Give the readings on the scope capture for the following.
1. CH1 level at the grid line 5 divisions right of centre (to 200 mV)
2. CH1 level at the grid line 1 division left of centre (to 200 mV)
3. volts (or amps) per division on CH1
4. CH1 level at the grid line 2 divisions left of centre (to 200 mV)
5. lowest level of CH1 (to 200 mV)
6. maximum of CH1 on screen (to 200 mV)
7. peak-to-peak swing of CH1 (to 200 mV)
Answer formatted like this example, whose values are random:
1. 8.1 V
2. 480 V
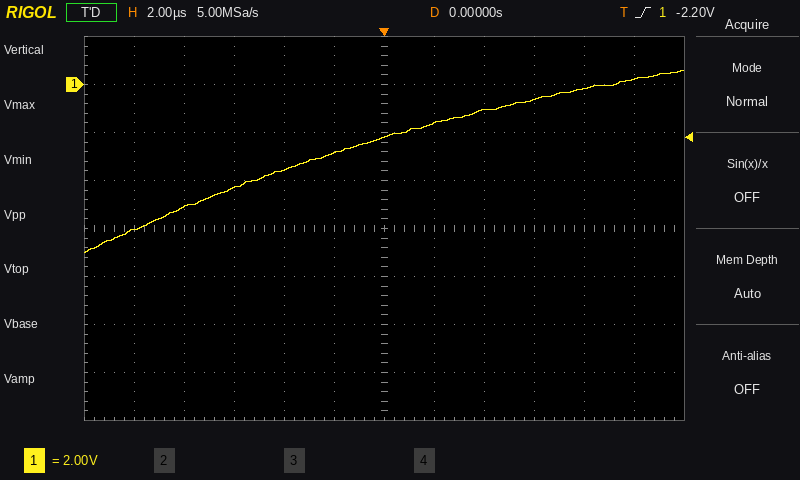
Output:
1. 200 mV
2. -2.8 V
3. 2 V
4. -3.6 V
5. -7.0 V
6. 600 mV
7. 7.6 V
